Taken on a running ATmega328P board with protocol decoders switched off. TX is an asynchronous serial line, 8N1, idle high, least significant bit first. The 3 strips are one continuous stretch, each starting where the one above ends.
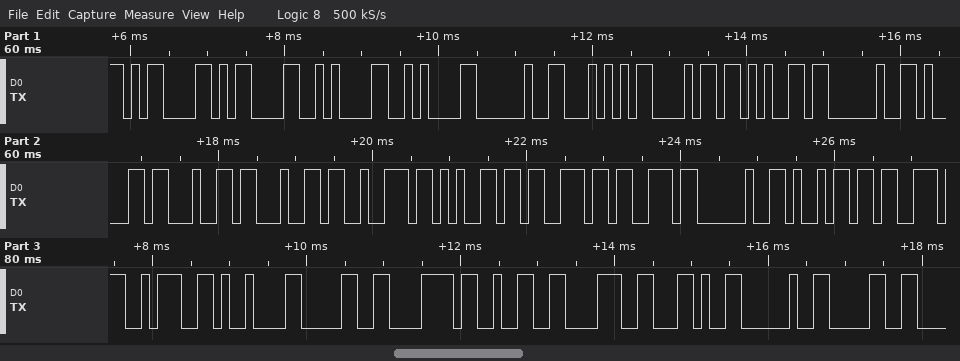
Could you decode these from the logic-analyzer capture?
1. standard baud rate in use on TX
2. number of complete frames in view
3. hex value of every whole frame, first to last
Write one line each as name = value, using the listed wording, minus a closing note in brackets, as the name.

standard baud rate in use on TX = 9600 baud
number of complete frames in view = 28
hex value of every whole frame, first to last = 0x0D 0x0D 0x0A 0x0A 0x20 0x54 0x68 0x65 0x20 0x61 0x64 0x64 0x72 0x65 0x73 0x73 0x20 0x69 0x73 0x3A 0x09 0x30 0x78 0x32 0x38 0x2C 0x20 0x30
